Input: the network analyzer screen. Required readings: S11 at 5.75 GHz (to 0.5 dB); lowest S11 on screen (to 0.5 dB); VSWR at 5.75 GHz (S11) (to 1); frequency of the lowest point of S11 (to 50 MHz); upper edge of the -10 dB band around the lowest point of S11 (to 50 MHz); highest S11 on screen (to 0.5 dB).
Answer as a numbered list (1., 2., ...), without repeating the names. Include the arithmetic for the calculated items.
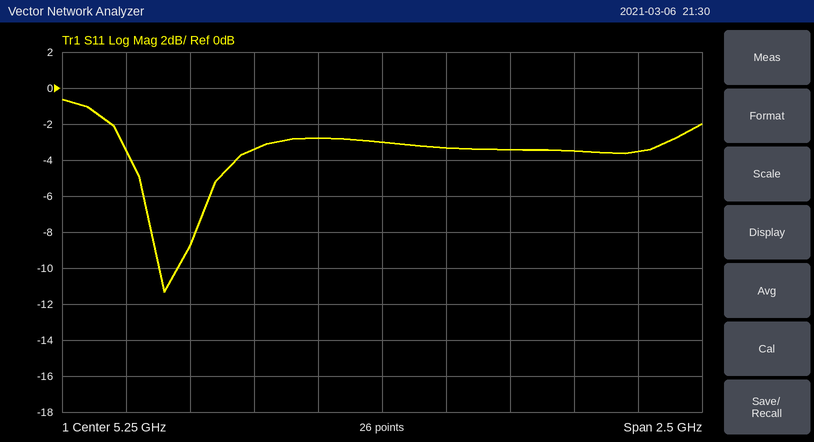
1. -3.5 dB
2. -11.5 dB
3. |Γ| = 10^(-3.5/20) = 0.6683; VSWR = (1 + 0.6683)/(1 − 0.6683) ≈ 5
4. 4.40 GHz
5. 4.45 GHz
6. -0.5 dB
